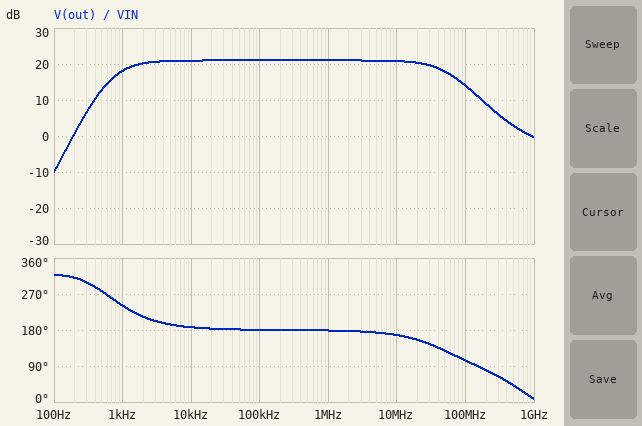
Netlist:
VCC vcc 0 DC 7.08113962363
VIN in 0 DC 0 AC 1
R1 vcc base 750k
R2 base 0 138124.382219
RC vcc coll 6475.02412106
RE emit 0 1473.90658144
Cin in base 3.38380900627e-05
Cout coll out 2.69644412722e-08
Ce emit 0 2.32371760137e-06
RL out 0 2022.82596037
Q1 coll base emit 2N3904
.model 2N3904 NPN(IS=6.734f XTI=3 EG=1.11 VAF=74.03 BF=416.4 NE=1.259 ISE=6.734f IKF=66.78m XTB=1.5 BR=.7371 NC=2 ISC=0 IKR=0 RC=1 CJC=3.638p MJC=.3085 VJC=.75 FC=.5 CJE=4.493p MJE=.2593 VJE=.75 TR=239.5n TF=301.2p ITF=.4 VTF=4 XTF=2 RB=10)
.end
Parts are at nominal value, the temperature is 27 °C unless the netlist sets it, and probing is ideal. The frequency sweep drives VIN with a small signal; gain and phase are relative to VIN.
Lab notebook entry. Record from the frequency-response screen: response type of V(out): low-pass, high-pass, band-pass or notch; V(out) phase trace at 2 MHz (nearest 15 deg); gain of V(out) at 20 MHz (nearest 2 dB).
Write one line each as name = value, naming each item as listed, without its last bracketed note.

response type of V(out): low-pass, high-pass, band-pass or notch = band-pass
V(out) phase trace at 2 MHz = 180 deg
gain of V(out) at 20 MHz = 20 dB
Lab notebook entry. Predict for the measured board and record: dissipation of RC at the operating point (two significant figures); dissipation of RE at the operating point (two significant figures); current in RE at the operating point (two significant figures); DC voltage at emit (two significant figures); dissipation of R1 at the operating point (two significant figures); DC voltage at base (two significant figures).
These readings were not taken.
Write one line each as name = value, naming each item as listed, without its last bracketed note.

dissipation of RC at the operating point = 230 µW
dissipation of RE at the operating point = 54 µW
current in RE at the operating point = 190 µA
DC voltage at emit = 280 mV
dissipation of R1 at the operating point = 51 µW
DC voltage at base = 900 mV
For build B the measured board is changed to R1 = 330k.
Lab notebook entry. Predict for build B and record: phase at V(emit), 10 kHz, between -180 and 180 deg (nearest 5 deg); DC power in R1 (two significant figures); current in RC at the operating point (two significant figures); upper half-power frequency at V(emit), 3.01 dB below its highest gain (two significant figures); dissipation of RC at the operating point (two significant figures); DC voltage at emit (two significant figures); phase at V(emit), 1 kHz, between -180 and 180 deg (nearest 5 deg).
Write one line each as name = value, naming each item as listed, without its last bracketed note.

phase at V(emit), 10 kHz, between -180 and 180 deg = -80 deg
DC power in R1 = 91 µW
current in RC at the operating point = 640 µA
upper half-power frequency at V(emit), 3.01 dB below its highest gain = 1.7 kHz
dissipation of RC at the operating point = 2.6 mW
DC voltage at emit = 950 mV
phase at V(emit), 1 kHz, between -180 and 180 deg = -30 deg
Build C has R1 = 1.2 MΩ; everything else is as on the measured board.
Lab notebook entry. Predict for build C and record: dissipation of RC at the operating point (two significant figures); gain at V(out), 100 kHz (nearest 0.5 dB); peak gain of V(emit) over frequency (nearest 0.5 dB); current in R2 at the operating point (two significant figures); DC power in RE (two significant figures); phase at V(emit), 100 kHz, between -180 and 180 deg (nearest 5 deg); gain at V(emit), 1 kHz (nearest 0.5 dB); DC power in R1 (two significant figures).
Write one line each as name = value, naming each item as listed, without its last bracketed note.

dissipation of RC at the operating point = 17 µW
gain at V(out), 100 kHz = 9.5 dB
peak gain of V(emit) over frequency = -2.5 dB
current in R2 at the operating point = 4.8 µA
DC power in RE = 3.9 µW
phase at V(emit), 100 kHz, between -180 and 180 deg = -90 deg
gain at V(emit), 1 kHz = -17.5 dB
DC power in R1 = 34 µW
